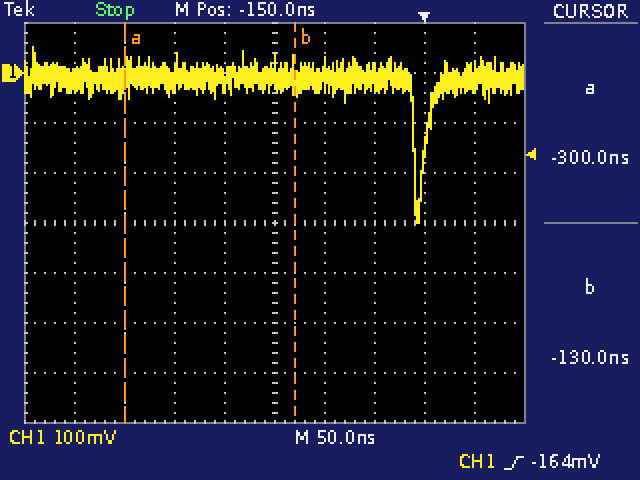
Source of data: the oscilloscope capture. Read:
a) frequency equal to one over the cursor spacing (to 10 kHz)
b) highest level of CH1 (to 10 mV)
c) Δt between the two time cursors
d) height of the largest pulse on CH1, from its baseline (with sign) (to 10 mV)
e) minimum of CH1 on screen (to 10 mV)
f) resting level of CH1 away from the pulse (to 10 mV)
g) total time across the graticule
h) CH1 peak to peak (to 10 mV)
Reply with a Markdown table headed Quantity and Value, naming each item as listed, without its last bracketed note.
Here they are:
| Quantity | Value |
|---|---|
| frequency equal to one over the cursor spacing | 5.88 MHz |
| highest level of CH1 | 50 mV |
| Δt between the two time cursors | 170 ns |
| height of the largest pulse on CH1, from its baseline (with sign) | -290 mV |
| minimum of CH1 on screen | -300 mV |
| resting level of CH1 away from the pulse | -10 mV |
| total time across the graticule | 500 ns |
| CH1 peak to peak | 350 mV |
